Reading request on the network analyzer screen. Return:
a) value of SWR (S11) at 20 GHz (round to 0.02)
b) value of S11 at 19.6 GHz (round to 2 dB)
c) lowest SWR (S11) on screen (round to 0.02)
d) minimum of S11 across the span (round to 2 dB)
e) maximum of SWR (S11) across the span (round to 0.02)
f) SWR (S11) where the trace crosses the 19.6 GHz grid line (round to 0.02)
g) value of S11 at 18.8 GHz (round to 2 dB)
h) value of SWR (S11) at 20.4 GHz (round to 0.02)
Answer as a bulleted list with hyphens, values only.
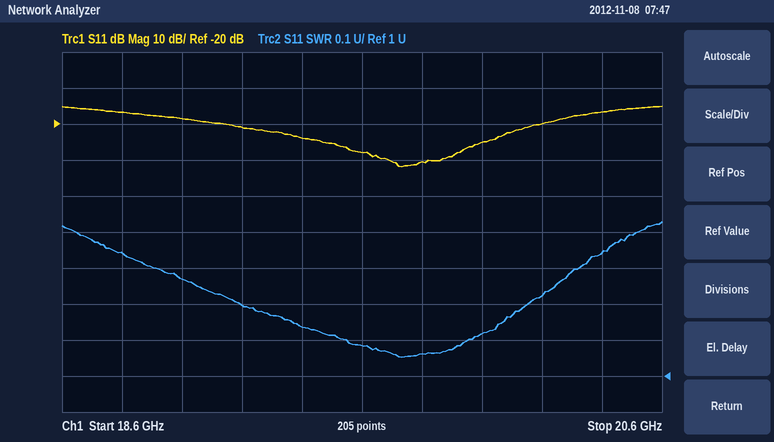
- 1.12
- -28 dB
- 1.06
- -32 dB
- 1.42
- 1.08
- -16 dB
- 1.34
